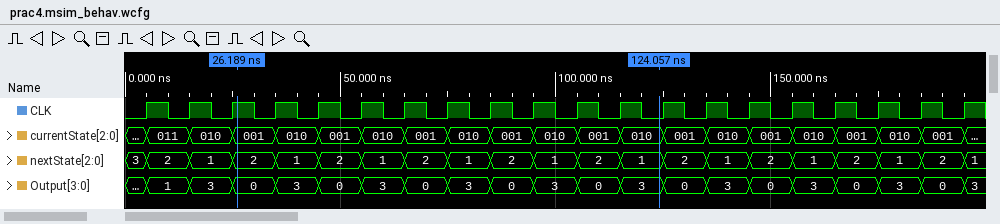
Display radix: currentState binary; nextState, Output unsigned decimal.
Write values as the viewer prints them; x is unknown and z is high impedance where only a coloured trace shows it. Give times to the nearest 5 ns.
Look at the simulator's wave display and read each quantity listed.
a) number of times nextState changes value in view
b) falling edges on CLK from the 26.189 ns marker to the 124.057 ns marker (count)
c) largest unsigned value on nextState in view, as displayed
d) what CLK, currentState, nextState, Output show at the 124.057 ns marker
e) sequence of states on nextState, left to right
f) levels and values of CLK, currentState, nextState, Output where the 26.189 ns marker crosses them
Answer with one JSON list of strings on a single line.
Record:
["20", "10", "3", "CLK=0, currentState=010, nextState=1, Output=3", "3, 2, 1, 2, 1, 2, 1, 2, 1, 2, 1, 2, 1, 2, 1, 2, 1, 2, 1, 2, 1", "CLK=1, currentState=001, nextState=2, Output=0"]
